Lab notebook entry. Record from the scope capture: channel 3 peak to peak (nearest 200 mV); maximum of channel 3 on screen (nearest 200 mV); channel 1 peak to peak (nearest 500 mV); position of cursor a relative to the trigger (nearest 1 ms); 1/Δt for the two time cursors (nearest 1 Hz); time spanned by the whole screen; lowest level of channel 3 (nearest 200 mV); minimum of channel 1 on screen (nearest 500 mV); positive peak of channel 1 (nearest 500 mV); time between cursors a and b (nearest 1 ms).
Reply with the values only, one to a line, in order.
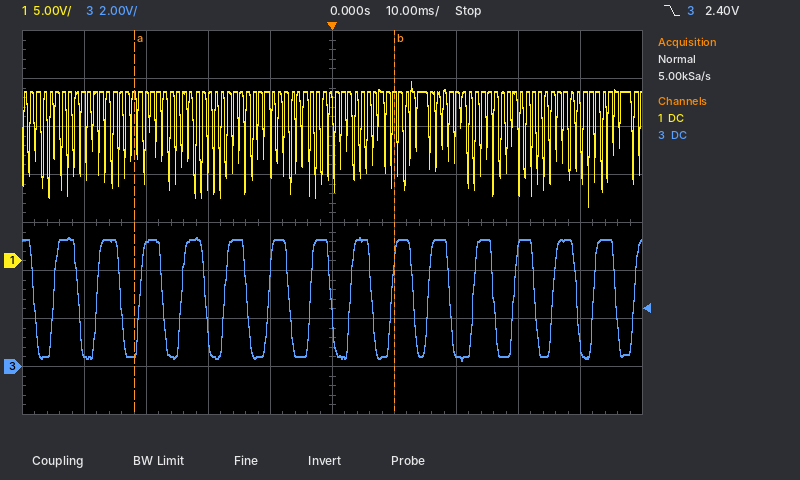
5.2 V
5.4 V
13.0 V
-32 ms
24 Hz
100 ms
200 mV
5.5 V
18.5 V
42 ms
